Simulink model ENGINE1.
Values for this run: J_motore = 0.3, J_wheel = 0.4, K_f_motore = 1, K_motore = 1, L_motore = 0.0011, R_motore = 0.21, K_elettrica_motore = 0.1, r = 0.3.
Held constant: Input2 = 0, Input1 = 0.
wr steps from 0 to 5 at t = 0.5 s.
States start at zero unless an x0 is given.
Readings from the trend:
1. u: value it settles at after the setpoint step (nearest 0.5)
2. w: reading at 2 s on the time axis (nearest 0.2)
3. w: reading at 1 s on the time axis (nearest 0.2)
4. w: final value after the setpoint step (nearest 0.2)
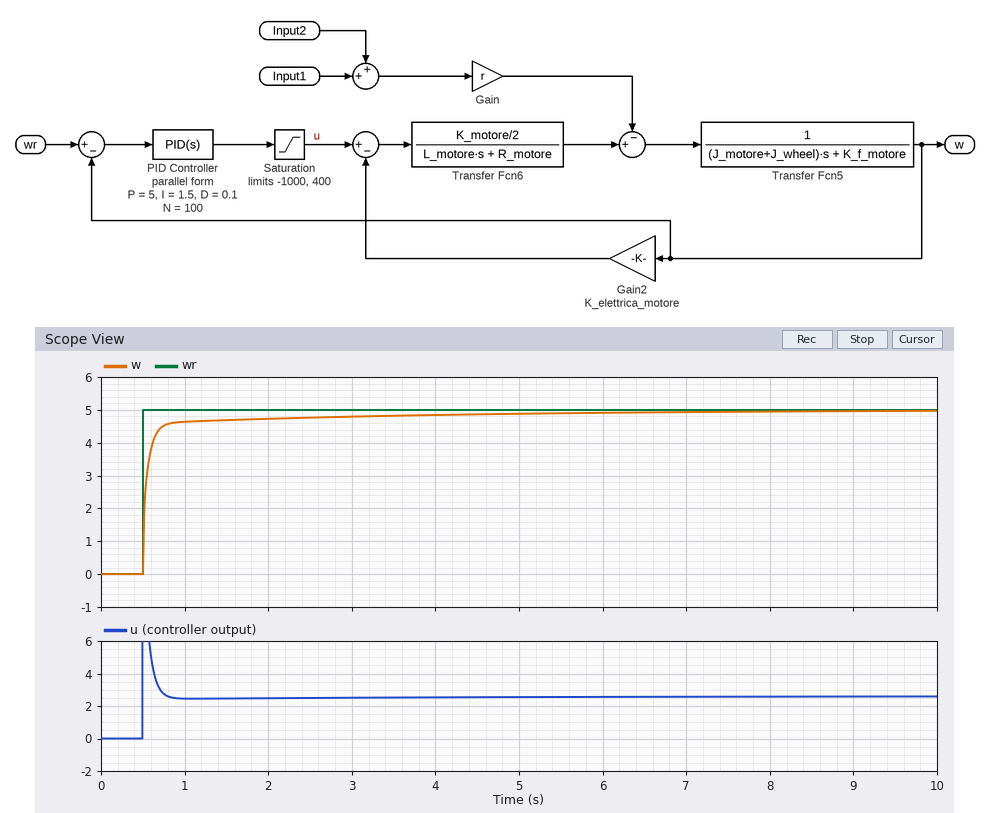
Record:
2.5
4.8
4.6
5.0
